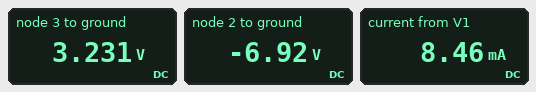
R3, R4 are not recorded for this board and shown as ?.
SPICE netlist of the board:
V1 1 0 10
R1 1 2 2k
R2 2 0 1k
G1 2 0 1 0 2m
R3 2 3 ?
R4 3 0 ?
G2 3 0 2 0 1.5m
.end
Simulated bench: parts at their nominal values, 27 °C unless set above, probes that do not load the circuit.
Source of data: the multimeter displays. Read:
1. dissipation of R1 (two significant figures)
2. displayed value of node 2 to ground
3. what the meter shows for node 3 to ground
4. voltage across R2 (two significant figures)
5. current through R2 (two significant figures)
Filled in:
140 mW
-6.92 V
3.231 V
6.9 V
6.9 mA
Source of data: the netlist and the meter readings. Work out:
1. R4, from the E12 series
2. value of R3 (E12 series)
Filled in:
560 Ω
2.2 kΩ
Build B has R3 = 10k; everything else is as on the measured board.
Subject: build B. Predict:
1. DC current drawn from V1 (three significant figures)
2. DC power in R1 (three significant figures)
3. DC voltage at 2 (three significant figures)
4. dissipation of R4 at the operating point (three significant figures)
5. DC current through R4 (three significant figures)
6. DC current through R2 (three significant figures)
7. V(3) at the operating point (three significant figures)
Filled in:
9.48 mA
180 mW
-8.96 V
79.0 mW
11.9 mA
8.96 mA
6.65 V
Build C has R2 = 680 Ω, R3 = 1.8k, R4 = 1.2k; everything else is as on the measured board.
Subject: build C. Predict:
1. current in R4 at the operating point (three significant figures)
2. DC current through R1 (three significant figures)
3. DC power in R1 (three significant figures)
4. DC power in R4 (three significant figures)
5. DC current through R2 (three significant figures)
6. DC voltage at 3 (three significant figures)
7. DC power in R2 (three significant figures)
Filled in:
2.93 mA
7.58 mA
115 mW
10.3 mW
7.60 mA
3.51 V
39.2 mW
